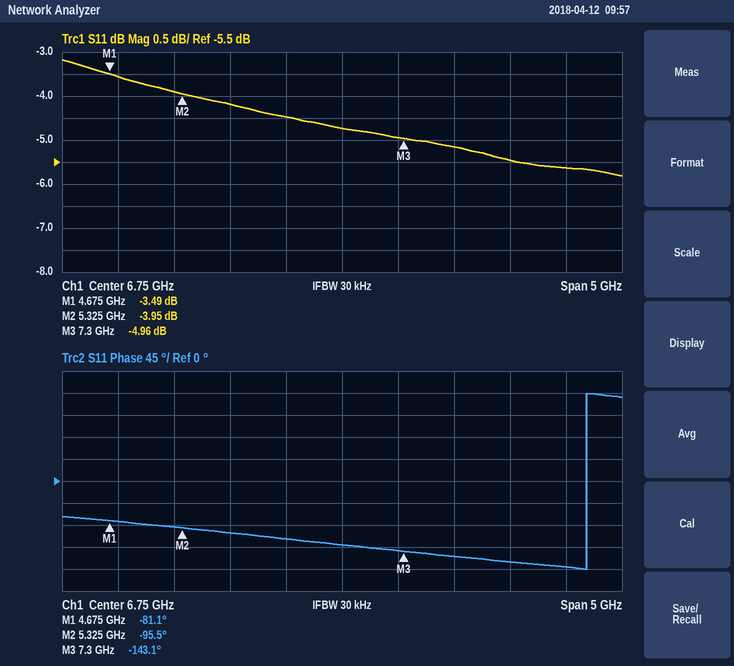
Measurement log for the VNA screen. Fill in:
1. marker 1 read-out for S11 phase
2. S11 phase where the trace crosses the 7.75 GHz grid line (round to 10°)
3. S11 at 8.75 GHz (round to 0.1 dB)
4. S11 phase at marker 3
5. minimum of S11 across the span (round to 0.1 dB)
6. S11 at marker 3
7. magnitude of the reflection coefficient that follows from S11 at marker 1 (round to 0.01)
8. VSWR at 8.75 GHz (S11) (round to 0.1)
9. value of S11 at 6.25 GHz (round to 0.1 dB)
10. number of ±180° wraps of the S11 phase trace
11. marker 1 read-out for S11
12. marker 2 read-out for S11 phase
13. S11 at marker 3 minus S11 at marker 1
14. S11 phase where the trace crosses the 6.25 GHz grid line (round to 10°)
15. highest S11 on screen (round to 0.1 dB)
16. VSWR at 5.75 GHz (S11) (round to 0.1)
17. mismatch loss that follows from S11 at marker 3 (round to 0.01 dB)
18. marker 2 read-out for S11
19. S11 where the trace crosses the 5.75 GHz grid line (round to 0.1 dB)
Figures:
-81.1°
-150°
-5.6 dB
-143.1°
-5.8 dB
-4.96 dB
0.67
3.2
-4.5 dB
1
-3.49 dB
-95.5°
-1.47 dB
-120°
-3.2 dB
4.2
1.67 dB
-3.95 dB
-4.2 dB
